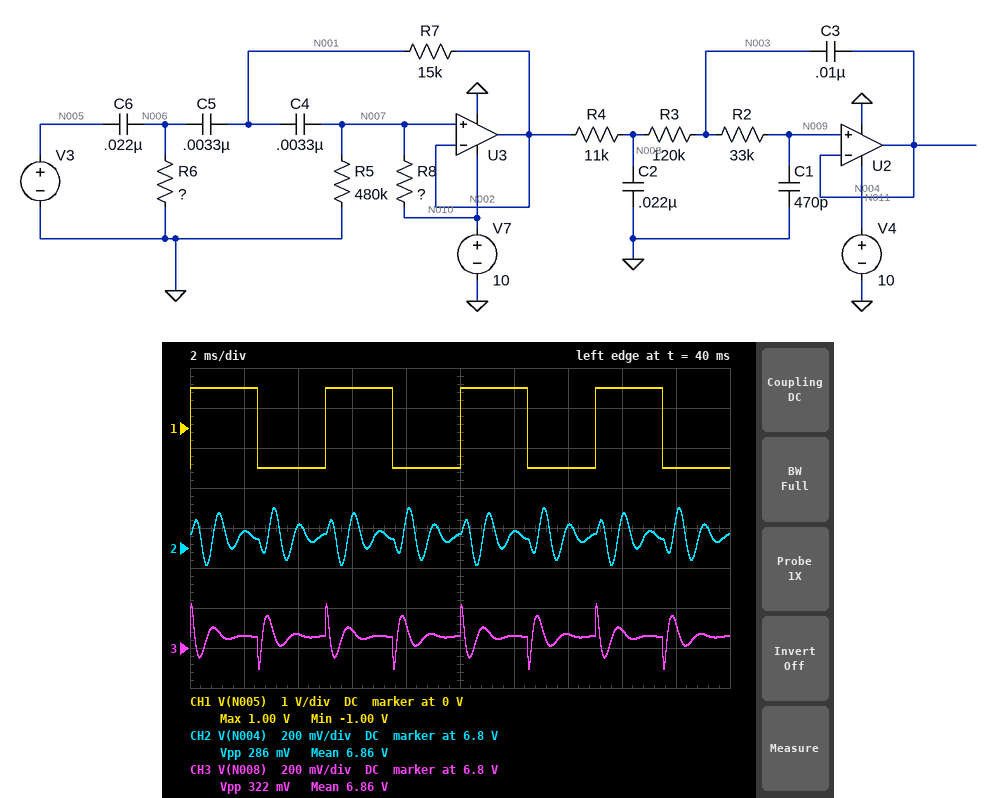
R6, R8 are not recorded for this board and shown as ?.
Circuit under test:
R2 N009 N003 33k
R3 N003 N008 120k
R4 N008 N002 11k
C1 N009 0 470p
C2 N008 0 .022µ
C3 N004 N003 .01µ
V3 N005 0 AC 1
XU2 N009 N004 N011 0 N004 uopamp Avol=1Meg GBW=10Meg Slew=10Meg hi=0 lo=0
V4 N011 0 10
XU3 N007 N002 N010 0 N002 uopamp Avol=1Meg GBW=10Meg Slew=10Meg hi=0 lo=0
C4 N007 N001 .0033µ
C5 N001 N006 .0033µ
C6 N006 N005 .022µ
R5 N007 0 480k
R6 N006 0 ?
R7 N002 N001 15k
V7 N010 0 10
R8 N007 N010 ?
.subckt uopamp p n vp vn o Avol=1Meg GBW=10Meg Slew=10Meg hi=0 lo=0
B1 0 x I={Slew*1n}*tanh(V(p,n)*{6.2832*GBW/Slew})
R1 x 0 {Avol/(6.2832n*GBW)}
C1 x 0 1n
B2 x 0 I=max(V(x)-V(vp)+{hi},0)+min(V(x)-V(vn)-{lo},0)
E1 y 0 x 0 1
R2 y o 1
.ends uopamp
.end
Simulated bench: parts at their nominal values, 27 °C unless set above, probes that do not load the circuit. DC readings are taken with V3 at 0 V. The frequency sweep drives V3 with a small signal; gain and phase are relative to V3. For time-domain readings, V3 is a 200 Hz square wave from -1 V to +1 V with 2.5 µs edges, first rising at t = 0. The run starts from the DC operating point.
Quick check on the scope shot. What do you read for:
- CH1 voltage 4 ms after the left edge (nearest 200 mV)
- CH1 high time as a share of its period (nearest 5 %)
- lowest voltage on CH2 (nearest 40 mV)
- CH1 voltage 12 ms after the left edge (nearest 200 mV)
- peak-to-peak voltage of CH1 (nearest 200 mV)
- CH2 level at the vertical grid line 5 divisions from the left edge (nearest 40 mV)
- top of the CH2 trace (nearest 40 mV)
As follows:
-1.0 V
50 %
6.72 V
1.0 V
2.0 V
6.88 V
7.00 V
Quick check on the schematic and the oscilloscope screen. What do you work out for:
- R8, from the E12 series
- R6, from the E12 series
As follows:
220 kΩ
1.5 kΩ
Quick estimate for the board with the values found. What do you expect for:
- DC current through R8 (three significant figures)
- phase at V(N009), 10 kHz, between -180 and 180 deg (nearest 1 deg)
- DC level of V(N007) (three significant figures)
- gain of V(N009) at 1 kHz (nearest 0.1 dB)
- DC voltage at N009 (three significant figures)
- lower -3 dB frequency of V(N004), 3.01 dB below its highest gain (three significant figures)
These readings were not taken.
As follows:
14.3 µA
127 deg
6.86 V
-10.5 dB
6.86 V
904 Hz
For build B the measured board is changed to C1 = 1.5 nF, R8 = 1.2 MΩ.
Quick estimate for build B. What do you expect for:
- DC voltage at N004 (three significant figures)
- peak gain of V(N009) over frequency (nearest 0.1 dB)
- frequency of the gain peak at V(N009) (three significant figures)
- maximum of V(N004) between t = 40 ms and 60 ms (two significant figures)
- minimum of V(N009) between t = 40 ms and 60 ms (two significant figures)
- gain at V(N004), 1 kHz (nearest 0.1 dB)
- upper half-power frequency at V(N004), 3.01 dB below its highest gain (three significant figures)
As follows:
2.86 V
-13.6 dB
681 Hz
3.0 V
2.8 V
-21.3 dB
828 Hz
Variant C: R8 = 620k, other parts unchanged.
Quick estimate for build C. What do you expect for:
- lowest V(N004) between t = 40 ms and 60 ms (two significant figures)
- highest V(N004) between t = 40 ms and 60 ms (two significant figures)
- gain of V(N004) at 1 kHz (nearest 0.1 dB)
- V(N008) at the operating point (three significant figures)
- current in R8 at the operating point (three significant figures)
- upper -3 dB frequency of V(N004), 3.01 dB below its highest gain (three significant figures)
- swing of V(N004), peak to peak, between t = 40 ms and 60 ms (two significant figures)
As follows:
4.2 V
4.5 V
-9.1 dB
4.36 V
9.09 µA
1.27 kHz
350 mV
